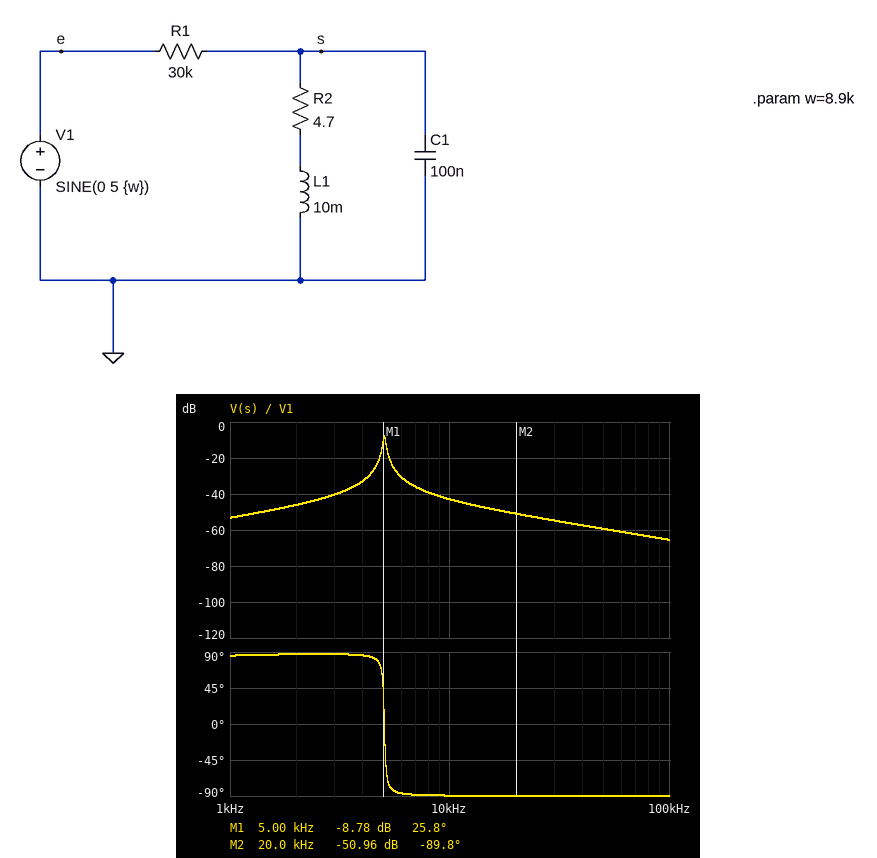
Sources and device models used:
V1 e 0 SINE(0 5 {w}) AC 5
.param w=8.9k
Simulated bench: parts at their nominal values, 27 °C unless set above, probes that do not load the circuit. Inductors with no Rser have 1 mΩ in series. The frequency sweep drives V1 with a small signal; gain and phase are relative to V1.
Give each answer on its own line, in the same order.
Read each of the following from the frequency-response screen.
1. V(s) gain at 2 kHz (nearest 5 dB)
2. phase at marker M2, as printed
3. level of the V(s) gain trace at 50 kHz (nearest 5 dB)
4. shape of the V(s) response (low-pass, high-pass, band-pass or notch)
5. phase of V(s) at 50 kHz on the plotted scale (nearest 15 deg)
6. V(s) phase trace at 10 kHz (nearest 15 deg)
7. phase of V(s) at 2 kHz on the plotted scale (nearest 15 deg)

-45 dB
-89.8 deg
-60 dB
band-pass
-90 deg
-90 deg
90 deg
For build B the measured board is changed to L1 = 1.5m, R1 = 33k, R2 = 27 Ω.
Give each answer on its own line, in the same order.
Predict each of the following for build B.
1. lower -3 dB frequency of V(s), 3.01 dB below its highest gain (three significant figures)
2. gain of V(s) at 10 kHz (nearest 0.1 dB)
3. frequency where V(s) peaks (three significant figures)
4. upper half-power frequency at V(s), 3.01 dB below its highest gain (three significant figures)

11.6 kHz
-43.5 dB
13.0 kHz
14.5 kHz
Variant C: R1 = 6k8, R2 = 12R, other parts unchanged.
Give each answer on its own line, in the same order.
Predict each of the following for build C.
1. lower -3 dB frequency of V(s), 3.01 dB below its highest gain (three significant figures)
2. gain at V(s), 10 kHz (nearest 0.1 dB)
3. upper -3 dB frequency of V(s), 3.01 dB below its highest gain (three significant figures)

4.83 kHz
-30.1 dB
5.25 kHz
